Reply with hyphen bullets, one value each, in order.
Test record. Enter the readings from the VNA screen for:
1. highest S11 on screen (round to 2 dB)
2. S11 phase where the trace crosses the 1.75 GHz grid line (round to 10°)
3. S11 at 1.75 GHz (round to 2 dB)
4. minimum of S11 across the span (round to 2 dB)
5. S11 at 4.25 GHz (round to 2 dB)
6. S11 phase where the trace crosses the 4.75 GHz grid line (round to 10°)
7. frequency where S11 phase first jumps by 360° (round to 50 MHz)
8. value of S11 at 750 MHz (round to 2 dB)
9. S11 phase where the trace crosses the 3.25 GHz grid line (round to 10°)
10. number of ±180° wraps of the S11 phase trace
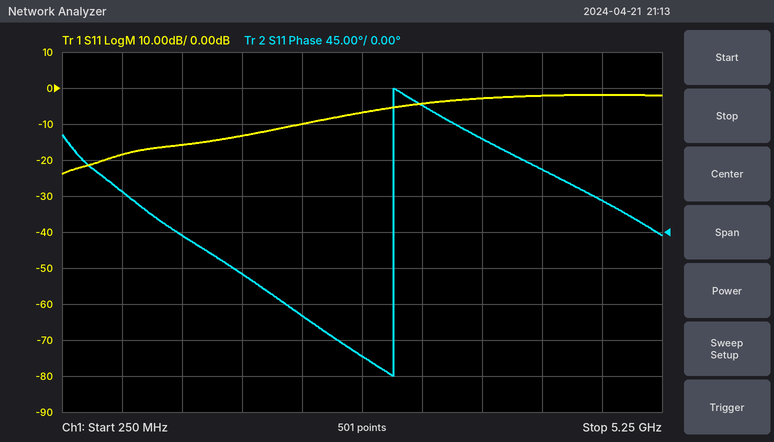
- -2 dB
- -50°
- -14 dB
- -24 dB
- -2 dB
- 40°
- 3.00 GHz
- -18 dB
- 160°
- 1
